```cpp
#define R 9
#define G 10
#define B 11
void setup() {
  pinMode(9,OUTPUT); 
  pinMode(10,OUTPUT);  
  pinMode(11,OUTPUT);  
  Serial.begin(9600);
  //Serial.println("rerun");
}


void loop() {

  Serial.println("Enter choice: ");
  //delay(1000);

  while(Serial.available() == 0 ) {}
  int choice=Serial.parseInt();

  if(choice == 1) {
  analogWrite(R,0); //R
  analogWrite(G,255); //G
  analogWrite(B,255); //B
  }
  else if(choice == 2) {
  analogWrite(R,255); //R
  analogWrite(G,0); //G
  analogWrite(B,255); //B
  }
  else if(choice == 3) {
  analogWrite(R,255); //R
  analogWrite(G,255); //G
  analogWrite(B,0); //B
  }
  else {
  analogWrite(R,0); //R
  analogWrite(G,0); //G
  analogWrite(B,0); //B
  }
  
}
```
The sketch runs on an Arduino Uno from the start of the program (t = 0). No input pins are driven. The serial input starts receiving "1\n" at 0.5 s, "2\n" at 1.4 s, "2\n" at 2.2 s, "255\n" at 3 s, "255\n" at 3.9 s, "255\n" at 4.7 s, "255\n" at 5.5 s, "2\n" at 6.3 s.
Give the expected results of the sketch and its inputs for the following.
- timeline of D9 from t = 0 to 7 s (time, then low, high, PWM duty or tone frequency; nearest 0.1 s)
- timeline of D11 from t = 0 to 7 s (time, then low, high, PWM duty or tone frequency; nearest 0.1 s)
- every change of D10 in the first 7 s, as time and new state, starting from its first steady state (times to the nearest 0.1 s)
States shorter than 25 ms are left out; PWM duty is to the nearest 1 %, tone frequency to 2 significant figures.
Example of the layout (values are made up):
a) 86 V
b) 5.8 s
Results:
a) 0 s low; 1.4 s high; 3 s low; 6.3 s high
b) 0 s low; 0.5 s high; 3 s low; 6.3 s high
c) 0 s low; 0.5 s high; 1.4 s low
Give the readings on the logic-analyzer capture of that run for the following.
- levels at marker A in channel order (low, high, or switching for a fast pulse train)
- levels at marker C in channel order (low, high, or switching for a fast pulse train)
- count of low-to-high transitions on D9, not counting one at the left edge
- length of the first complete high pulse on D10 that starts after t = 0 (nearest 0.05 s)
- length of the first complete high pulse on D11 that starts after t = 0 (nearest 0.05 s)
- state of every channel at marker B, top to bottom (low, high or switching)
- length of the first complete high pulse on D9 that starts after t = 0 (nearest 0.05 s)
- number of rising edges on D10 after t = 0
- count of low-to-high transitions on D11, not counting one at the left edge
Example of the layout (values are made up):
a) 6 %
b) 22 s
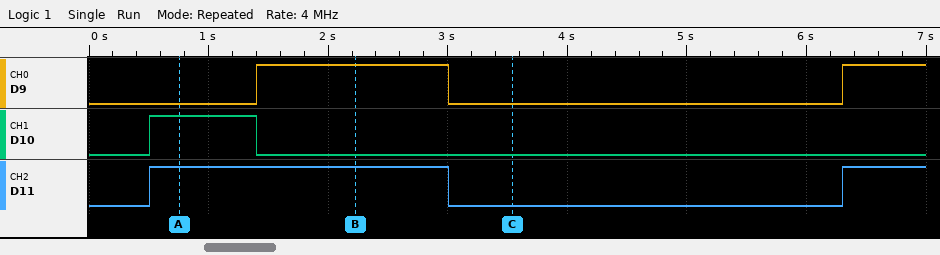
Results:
a) D9 low, D10 high, D11 high
b) D9 low, D10 low, D11 low
c) 2
d) 0.90 s
e) 2.50 s
f) D9 high, D10 low, D11 high
g) 1.60 s
h) 1
i) 2
